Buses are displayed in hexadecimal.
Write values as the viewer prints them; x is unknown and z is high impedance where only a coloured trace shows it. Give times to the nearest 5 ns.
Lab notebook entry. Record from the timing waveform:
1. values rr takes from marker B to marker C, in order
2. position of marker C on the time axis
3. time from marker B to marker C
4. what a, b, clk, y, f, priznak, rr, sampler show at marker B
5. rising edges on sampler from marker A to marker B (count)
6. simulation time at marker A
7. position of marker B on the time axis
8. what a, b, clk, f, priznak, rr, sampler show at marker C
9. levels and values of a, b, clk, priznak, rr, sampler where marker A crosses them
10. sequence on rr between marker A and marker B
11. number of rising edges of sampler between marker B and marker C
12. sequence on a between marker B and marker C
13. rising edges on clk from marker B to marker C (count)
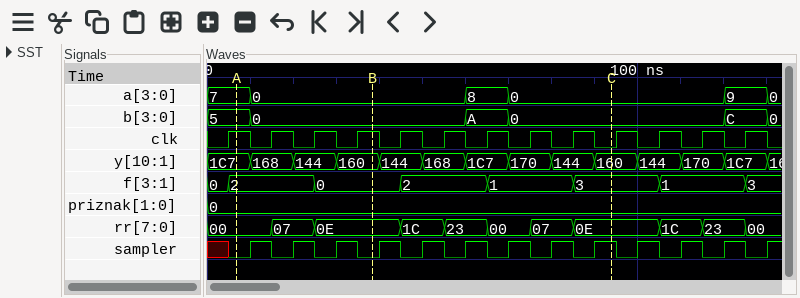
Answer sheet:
0E, 1C, 23, 00, 07, 0E
95 ns
55 ns
a=0, b=0, clk=1, y=160, f=0, priznak=0, rr=0E, sampler=0
3
5 ns
40 ns
a=0, b=0, clk=0, f=3, priznak=0, rr=0E, sampler=1
a=7, b=5, clk=1, priznak=0, rr=00, sampler=0
00, 07, 0E
6
0, 8, 0
5
